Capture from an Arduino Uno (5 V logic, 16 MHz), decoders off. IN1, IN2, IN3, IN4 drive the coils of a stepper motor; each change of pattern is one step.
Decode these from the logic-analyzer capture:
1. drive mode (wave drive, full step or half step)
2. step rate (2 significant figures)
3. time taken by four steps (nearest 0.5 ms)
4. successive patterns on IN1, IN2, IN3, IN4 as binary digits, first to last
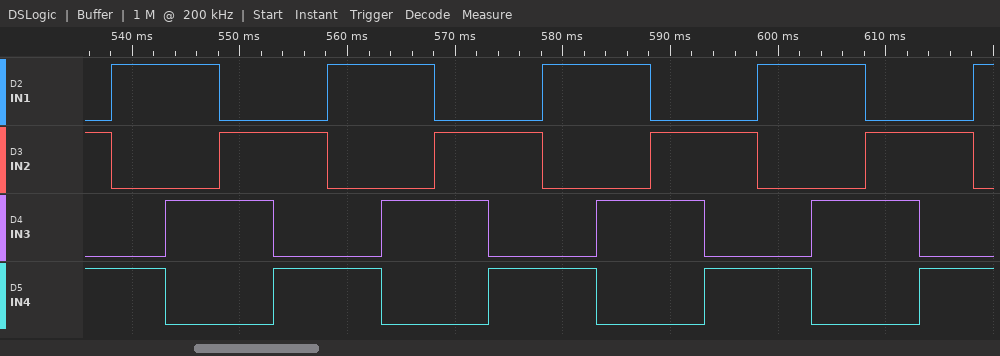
full step
200 steps/s
20.0 ms
0101 1001 1010 0110 0101 1001 1010 0110 0101 1001 1010 0110 0101 1001 1010 0110 0101 1001
